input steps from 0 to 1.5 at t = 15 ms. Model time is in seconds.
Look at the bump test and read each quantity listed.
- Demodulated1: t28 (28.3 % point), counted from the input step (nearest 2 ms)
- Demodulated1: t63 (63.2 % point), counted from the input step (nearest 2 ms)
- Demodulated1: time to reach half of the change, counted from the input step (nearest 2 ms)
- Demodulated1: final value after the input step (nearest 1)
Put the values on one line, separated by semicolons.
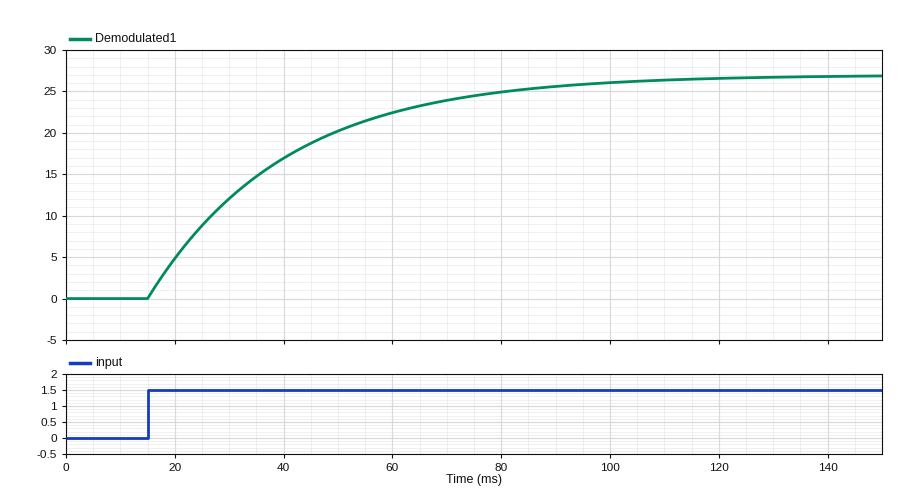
8 ms; 26 ms; 18 ms; 27
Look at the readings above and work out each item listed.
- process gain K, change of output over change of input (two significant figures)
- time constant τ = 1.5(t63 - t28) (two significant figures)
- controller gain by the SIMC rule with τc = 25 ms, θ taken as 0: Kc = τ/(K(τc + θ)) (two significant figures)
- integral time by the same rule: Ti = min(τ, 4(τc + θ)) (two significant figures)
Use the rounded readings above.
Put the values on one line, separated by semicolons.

18; 27 ms; 0.060; 27 ms
